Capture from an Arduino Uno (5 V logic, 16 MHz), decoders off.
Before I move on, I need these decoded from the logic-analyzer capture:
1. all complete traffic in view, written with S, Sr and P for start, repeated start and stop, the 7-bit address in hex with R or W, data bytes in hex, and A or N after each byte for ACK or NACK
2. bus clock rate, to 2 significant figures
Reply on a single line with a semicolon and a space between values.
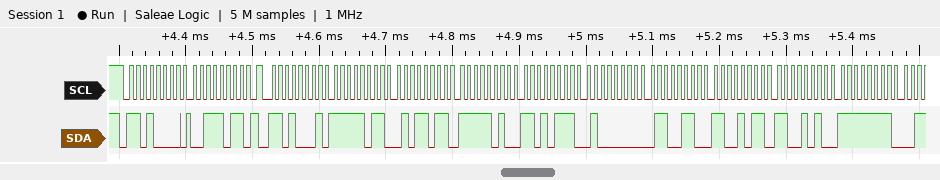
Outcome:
S 68W A 3B A Sr 68R A FB A 5B A FA A D7 A 40 A 66 A CB A CA A FF A; 100 kHz
